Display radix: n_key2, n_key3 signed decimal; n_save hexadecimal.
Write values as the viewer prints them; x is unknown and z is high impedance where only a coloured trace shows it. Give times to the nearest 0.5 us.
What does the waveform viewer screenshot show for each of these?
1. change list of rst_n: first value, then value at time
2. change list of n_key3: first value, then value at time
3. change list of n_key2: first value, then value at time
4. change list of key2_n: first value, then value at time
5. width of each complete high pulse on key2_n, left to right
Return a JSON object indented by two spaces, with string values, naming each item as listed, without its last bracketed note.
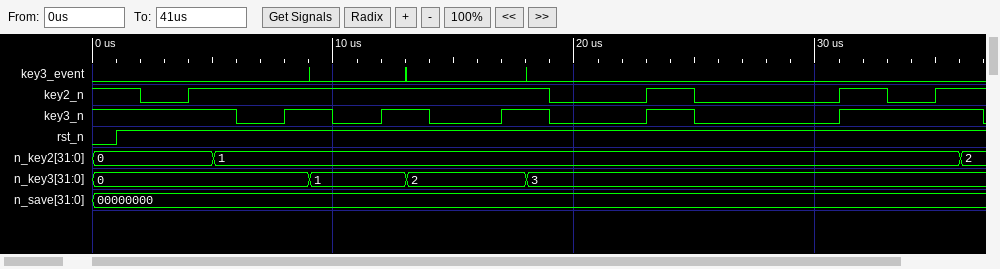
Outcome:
{
  "change list of rst_n: first value, then value at time": "0, 1 at 1 us",
  "change list of n_key3: first value, then value at time": "0, 1 at 9 us, 2 at 13 us, 3 at 18 us",
  "change list of n_key2: first value, then value at time": "0, 1 at 5 us, 2 at 36 us",
  "change list of key2_n: first value, then value at time": "1, 0 at 2 us, 1 at 4 us, 0 at 19 us, 1 at 23 us, 0 at 25 us, 1 at 31 us, 0 at 33 us, 1 at 35 us",
  "width of each complete high pulse on key2_n, left to right": "15 us, 2 us, 2 us"
}
